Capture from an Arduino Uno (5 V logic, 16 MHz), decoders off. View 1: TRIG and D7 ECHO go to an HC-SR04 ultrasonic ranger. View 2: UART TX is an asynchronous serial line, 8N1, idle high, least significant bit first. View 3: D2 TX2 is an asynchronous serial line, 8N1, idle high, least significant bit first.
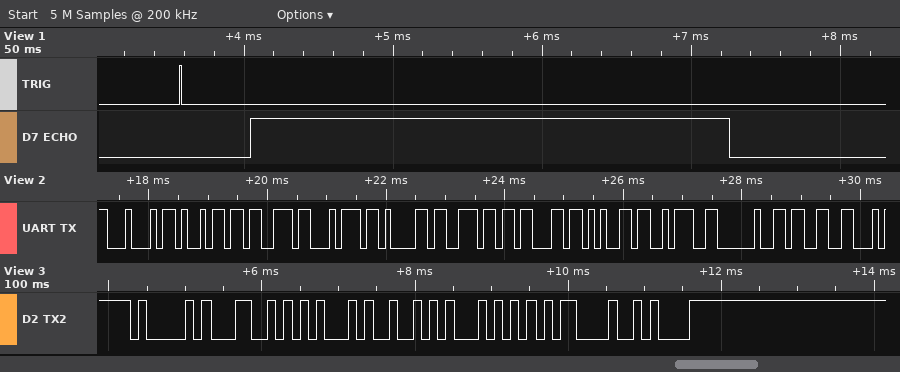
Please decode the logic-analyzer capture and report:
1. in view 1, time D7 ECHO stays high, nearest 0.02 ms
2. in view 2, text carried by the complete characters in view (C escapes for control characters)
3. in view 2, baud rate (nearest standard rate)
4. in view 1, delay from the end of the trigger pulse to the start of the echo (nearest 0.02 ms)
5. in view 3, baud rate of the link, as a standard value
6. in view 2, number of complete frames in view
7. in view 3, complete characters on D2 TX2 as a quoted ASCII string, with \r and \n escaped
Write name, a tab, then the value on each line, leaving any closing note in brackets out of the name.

in view 1, time D7 ECHO stays high, nearest 0.02 ms	3.22 ms
in view 2, text carried by the complete characters in view	"Distance: 3"
in view 2, baud rate	9600 baud
in view 1, delay from the end of the trigger pulse to the start of the echo	0.46 ms
in view 3, baud rate of the link, as a standard value	9600 baud
in view 2, number of complete frames in view	11
in view 3, complete characters on D2 TX2 as a quoted ASCII string, with \r and \n escaped	"ALERT\r\n"
